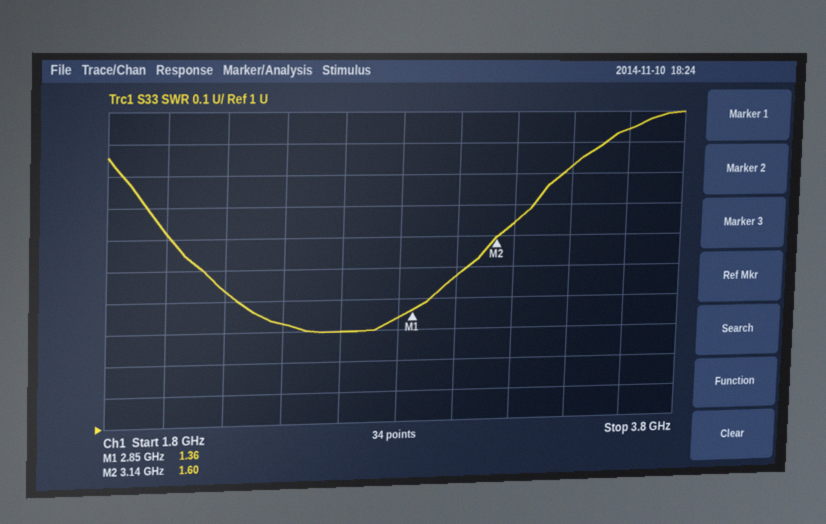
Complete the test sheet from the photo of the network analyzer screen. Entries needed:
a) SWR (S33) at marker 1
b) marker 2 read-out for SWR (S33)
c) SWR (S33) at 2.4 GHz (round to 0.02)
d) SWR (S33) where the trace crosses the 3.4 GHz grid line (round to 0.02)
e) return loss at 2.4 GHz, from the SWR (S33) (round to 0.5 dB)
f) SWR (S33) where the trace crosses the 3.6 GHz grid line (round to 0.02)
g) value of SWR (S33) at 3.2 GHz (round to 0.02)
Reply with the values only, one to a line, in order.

1.36
1.60
1.32
1.82
17.0 dB
1.94
1.64
